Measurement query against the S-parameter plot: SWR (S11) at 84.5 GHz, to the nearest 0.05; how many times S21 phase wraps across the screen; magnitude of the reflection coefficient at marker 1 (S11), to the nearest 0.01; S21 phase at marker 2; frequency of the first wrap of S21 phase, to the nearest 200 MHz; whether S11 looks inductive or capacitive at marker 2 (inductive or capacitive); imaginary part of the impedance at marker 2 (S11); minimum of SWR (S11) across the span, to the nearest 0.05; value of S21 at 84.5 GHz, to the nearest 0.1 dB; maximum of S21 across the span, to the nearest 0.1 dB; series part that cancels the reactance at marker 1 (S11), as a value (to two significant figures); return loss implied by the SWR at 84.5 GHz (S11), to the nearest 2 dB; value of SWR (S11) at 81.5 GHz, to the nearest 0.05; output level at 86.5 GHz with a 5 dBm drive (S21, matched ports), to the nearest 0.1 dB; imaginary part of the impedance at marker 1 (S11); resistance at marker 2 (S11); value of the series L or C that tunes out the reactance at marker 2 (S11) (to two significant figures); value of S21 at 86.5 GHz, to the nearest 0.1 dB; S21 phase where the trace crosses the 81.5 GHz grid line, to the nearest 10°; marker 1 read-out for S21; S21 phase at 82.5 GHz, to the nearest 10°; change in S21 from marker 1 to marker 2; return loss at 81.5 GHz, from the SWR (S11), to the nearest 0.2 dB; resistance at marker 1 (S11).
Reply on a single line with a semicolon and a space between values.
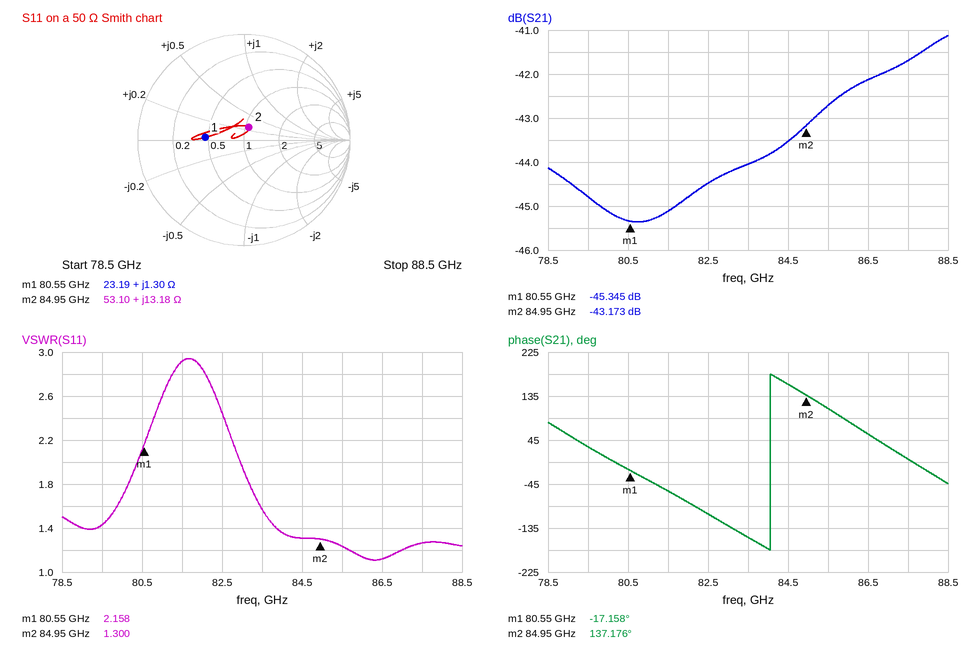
1.30; 1; 0.37; 137.176°; 84.0 GHz; inductive; +13.18 Ω; 1.10; -43.5 dB; -41.1 dB; 1.5 pF; 18 dB; 2.90; -37.1 dBm; +1.30 Ω; 53.10 Ω; 140 fF; -42.1 dB; -60°; -45.345 dB; -110°; 2.172 dB; 6.2 dB; 23.19 Ω
